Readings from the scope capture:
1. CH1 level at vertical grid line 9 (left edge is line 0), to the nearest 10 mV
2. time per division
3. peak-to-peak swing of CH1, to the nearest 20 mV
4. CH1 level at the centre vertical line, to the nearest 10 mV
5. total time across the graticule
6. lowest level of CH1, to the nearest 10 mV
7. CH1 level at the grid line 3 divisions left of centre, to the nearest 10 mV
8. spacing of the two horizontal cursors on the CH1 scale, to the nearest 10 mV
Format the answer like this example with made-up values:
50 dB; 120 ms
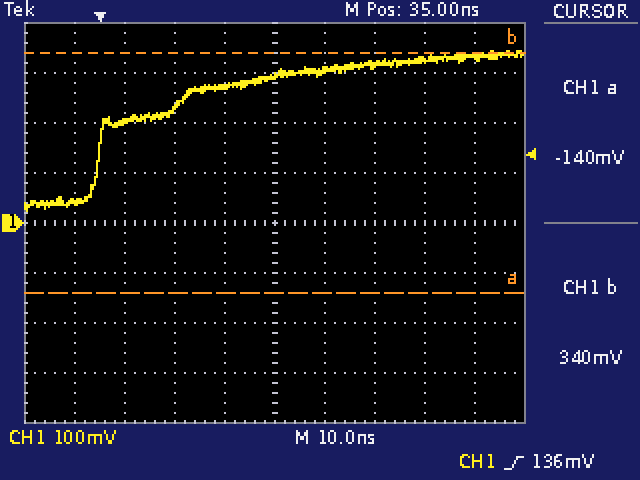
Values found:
330 mV; 10 ns; 320 mV; 290 mV; 100 ns; 20 mV; 200 mV; 480 mV
